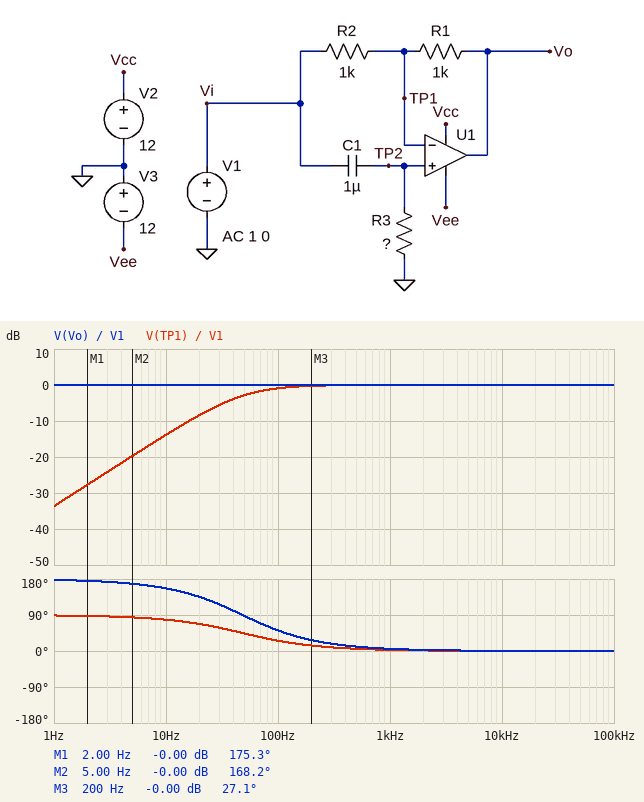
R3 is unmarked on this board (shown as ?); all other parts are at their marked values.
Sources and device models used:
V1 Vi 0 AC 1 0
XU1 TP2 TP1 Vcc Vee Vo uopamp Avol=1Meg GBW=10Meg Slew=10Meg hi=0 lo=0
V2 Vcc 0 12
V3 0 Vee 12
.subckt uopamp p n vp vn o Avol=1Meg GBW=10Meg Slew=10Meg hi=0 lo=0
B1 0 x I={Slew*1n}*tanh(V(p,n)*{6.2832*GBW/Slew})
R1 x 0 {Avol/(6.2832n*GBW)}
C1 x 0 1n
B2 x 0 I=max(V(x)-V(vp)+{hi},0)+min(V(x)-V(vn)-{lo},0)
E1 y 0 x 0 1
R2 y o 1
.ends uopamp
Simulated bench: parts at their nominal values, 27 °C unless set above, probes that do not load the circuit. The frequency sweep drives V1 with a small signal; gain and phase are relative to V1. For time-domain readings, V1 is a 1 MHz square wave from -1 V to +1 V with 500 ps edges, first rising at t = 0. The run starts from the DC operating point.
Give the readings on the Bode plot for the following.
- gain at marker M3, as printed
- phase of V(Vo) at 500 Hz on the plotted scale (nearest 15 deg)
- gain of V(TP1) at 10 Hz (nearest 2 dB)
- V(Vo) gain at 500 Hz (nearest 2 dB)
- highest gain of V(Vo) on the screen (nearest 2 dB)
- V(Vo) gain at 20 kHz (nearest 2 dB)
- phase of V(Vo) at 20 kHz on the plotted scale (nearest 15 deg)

-0.00 dB
15 deg
-14 dB
0 dB
0 dB
0 dB
0 deg
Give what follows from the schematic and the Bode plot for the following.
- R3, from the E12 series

3.3 kΩ
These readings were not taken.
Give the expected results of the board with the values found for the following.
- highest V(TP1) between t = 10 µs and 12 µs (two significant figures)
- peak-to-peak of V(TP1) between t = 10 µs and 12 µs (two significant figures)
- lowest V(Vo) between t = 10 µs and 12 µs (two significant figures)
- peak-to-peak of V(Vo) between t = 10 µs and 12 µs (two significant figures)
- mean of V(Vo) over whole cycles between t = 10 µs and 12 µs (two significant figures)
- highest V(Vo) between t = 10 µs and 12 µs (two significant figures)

2.0 V
2.0 V
990 mV
2.0 V
2.0 V
3.0 V
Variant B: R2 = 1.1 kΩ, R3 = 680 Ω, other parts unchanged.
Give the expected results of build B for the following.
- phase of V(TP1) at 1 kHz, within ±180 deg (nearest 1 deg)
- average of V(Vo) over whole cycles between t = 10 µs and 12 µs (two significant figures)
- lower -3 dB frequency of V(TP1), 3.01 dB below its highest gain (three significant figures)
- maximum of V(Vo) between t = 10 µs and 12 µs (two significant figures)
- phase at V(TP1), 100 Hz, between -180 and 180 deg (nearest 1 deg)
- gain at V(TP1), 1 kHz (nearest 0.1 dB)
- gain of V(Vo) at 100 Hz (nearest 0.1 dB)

13 deg
1.9 V
234 Hz
2.9 V
67 deg
-0.2 dB
-0.7 dB
